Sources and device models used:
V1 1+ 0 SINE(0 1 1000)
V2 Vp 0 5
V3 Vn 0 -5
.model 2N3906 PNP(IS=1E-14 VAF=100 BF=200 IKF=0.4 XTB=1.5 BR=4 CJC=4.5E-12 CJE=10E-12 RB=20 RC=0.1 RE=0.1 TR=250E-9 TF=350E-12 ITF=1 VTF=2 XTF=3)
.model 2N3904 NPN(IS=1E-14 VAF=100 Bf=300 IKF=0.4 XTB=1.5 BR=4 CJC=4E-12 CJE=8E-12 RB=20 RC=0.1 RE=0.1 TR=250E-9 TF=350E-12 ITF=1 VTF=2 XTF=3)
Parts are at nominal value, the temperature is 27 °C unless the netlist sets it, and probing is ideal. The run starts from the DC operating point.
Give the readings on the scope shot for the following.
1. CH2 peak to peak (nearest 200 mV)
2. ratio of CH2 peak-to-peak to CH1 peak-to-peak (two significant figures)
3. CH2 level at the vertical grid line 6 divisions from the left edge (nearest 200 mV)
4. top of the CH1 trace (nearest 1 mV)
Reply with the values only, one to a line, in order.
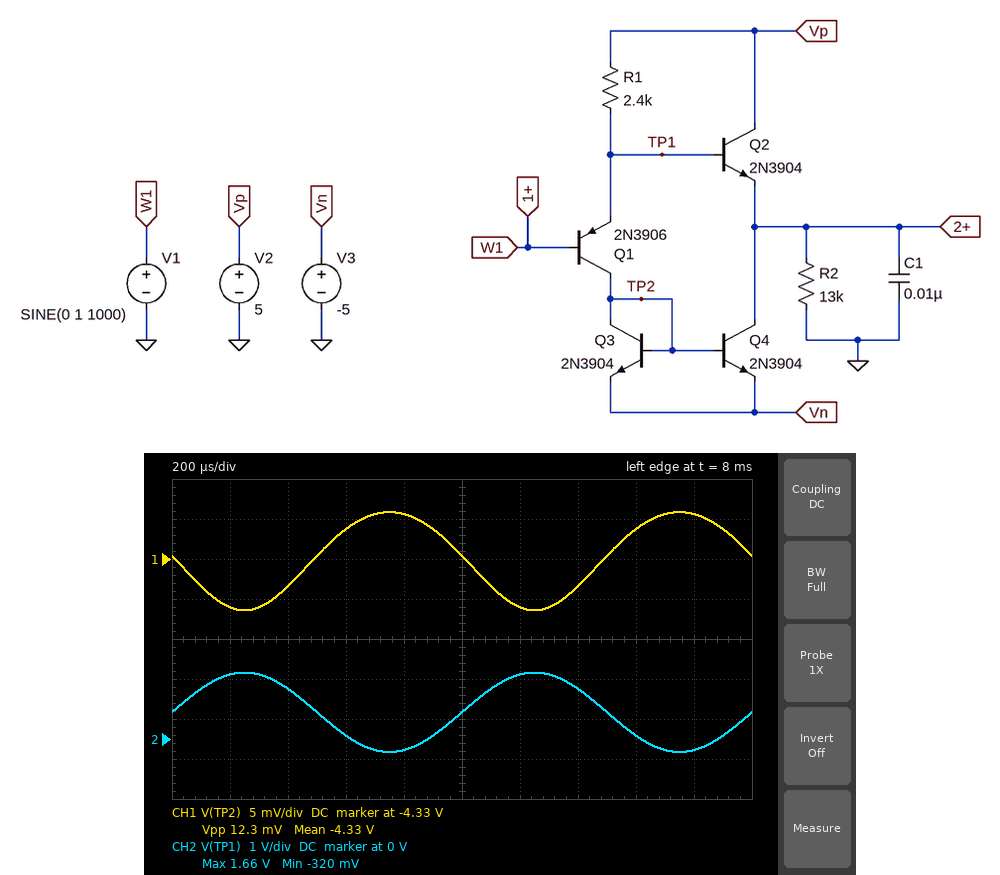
2.0 V
160
1.6 V
-4.324 V
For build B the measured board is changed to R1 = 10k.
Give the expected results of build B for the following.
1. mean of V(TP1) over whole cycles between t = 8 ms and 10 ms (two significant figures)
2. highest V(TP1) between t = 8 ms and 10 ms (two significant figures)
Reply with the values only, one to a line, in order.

630 mV
1.6 V
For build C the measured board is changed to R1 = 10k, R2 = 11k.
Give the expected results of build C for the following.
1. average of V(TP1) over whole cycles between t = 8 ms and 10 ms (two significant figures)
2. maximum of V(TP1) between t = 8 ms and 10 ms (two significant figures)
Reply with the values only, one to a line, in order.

630 mV
1.6 V
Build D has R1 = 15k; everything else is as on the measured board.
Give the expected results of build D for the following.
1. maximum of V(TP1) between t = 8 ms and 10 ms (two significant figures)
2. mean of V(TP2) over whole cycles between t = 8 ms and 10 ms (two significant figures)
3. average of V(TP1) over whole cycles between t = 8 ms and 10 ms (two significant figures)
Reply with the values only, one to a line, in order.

1.6 V
-4.4 V
620 mV
